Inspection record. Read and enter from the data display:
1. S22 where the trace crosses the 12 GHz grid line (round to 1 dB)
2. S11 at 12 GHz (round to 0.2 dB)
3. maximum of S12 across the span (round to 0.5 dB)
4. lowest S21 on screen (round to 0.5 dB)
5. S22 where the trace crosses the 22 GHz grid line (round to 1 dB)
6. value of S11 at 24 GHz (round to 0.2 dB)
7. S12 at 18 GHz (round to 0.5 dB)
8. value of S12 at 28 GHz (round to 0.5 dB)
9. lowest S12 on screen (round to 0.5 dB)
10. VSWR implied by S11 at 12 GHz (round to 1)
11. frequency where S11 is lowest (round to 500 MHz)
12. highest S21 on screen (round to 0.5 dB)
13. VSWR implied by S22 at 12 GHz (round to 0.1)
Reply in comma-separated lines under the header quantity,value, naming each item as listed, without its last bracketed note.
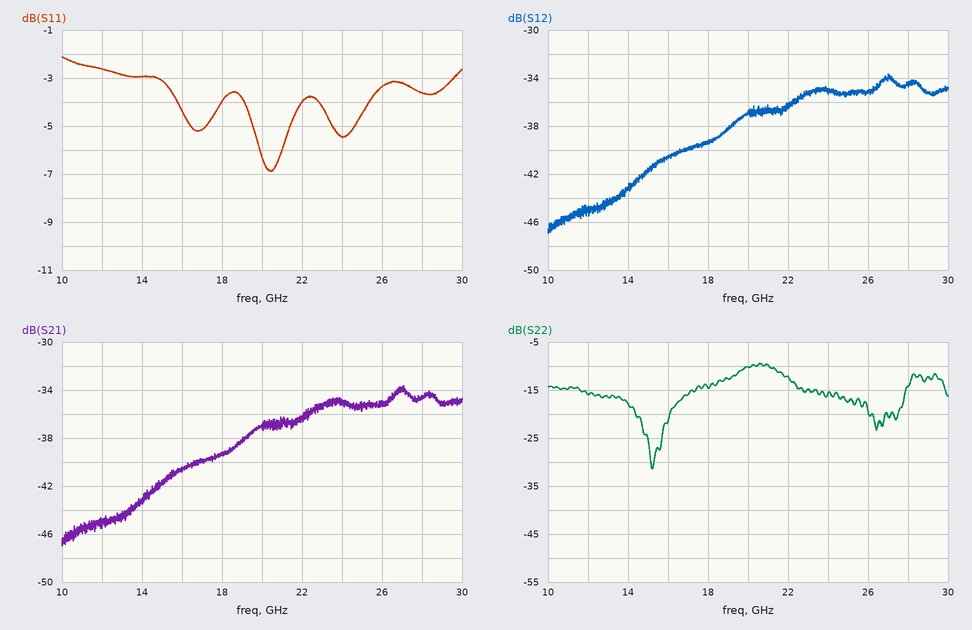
quantity,value
S22 where the trace crosses the 12 GHz grid line,-16 dB
S11 at 12 GHz,-2.6 dB
maximum of S12 across the span,-33.5 dB
lowest S21 on screen,-47.0 dB
S22 where the trace crosses the 22 GHz grid line,-12 dB
value of S11 at 24 GHz,-5.4 dB
S12 at 18 GHz,-39.5 dB
value of S12 at 28 GHz,-34.5 dB
lowest S12 on screen,-47.0 dB
VSWR implied by S11 at 12 GHz,7
frequency where S11 is lowest,20.5 GHz
highest S21 on screen,-33.5 dB
VSWR implied by S22 at 12 GHz,1.4
